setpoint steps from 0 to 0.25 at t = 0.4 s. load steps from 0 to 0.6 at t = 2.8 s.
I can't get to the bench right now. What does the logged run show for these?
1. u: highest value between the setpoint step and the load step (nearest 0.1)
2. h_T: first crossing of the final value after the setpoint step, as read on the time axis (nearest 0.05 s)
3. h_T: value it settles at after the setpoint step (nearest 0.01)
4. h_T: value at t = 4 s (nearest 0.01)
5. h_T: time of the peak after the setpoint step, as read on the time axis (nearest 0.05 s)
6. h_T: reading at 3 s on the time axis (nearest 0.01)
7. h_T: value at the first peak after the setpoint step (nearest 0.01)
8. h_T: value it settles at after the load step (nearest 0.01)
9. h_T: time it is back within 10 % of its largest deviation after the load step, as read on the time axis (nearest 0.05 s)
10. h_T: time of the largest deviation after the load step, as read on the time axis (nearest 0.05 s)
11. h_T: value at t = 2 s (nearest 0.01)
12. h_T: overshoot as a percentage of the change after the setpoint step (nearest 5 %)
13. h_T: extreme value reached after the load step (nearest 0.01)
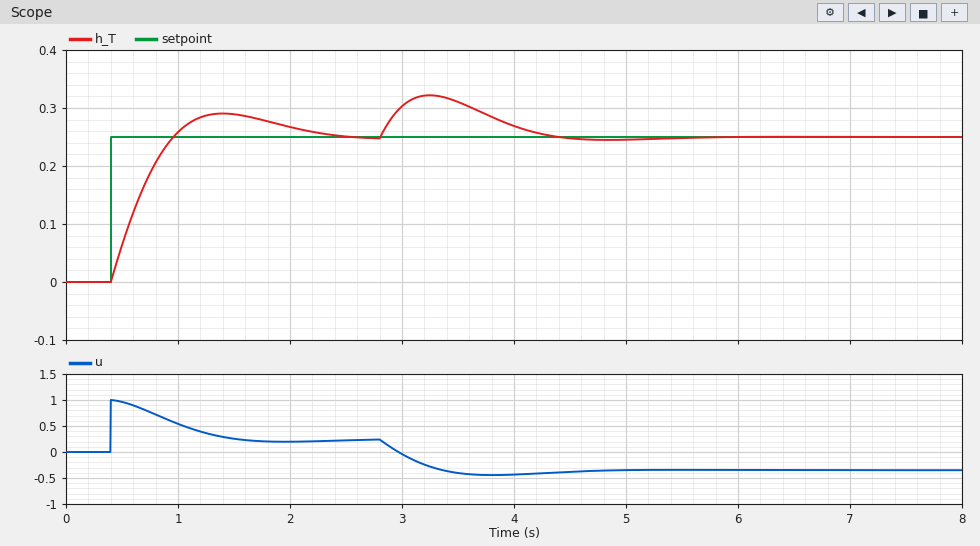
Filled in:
1.0
0.95 s
0.25
0.27
1.40 s
0.30
0.29
0.25
4.20 s
3.25 s
0.27
15 %
0.32
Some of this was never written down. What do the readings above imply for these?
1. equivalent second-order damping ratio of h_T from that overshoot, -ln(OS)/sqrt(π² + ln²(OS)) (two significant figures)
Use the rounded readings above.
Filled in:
0.52
